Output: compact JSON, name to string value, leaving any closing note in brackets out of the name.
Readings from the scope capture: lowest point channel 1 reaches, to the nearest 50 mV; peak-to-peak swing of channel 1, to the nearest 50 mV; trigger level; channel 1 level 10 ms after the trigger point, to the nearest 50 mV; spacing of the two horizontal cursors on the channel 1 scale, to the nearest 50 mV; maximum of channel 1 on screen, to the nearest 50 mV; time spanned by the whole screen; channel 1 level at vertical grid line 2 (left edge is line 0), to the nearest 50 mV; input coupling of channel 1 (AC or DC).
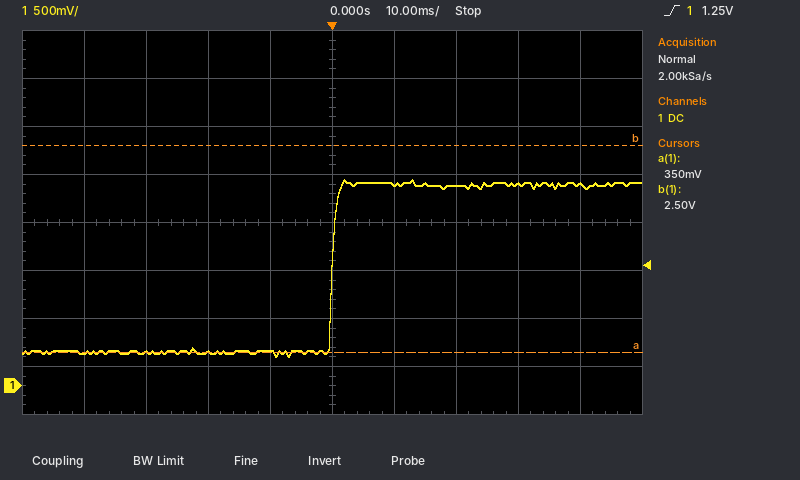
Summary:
{"lowest point channel 1 reaches, to the nearest 50 mV": "300 mV", "peak-to-peak swing of channel 1, to the nearest 50 mV": "1.85 V", "trigger level": "1.25 V", "channel 1 level 10 ms after the trigger point, to the nearest 50 mV": "2.10 V", "spacing of the two horizontal cursors on the channel 1 scale, to the nearest 50 mV": "2.15 V", "maximum of channel 1 on screen, to the nearest 50 mV": "2.15 V", "time spanned by the whole screen": "100 ms", "channel 1 level at vertical grid line 2 (left edge is line 0), to the nearest 50 mV": "350 mV", "input coupling of channel 1": "DC"}
